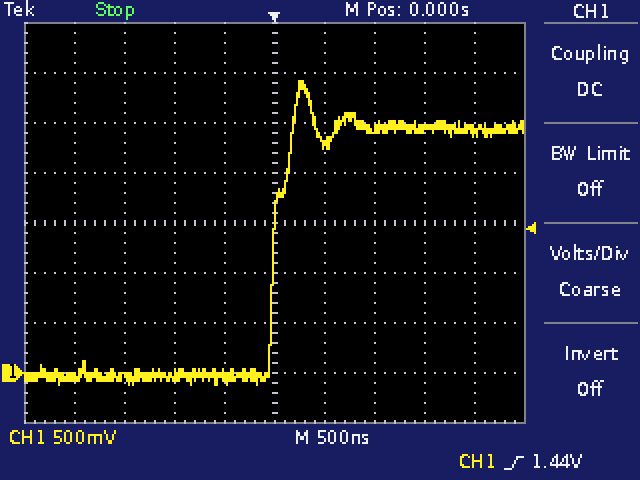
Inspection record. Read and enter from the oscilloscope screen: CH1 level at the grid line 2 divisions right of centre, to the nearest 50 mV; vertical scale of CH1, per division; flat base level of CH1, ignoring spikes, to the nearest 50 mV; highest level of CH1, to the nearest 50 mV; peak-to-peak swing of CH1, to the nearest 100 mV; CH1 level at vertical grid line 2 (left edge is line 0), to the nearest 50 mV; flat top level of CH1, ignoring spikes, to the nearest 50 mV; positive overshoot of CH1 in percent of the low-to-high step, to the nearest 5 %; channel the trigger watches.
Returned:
2.45 V
500 mV
-50 mV
2.90 V
3.00 V
-50 mV
2.45 V
20 %
CH1
